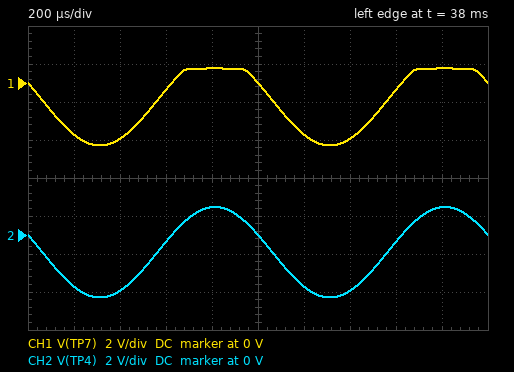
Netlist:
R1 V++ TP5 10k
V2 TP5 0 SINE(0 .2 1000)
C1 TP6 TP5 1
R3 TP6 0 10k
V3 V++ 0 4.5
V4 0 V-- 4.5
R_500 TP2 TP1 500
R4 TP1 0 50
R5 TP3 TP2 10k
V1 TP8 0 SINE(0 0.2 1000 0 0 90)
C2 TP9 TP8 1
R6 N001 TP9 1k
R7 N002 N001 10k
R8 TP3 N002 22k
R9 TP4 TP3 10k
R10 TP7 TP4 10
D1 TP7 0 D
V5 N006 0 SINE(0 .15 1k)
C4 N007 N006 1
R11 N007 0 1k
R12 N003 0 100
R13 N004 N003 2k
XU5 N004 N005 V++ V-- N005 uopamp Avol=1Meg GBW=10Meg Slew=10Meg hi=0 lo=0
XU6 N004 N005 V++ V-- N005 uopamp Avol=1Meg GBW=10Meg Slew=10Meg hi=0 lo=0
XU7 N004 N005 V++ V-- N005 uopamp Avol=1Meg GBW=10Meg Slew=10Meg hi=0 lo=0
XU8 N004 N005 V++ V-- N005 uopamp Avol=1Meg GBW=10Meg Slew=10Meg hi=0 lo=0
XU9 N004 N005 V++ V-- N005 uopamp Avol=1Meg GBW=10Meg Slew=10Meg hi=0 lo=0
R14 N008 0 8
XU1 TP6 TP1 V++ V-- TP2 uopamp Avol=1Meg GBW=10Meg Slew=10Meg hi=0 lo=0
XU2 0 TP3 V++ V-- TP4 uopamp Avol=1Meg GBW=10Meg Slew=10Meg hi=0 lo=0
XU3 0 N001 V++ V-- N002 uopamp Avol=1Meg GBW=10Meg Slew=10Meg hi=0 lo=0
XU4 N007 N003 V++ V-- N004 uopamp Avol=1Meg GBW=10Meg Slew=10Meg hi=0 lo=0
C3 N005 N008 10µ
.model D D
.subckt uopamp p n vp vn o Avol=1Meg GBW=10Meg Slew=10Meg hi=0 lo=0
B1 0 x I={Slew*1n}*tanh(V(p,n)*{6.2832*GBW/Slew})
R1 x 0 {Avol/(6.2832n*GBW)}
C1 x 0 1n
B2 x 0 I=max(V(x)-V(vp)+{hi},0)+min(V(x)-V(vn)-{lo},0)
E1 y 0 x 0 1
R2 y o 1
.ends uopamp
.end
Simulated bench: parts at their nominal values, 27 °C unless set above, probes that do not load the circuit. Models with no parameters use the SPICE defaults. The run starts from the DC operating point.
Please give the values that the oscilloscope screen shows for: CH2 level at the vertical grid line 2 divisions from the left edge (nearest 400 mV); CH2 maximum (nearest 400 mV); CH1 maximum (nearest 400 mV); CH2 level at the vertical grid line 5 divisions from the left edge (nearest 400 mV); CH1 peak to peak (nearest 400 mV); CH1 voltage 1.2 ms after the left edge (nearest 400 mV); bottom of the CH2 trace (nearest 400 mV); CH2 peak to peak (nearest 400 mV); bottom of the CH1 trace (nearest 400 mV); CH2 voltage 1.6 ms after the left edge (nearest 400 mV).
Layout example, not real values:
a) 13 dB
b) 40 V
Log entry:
a) -2.8 V
b) 1.6 V
c) 800 mV
d) 0 V
e) 4.0 V
f) -2.8 V
g) -3.2 V
h) 4.8 V
i) -3.2 V
j) -400 mV
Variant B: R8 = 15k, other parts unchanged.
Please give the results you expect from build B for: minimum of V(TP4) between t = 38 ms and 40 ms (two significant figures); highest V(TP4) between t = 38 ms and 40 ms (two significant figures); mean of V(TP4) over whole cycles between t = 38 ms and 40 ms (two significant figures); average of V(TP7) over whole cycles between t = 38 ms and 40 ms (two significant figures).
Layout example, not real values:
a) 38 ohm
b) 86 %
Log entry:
a) -3.9 V
b) 1.2 V
c) -1.3 V
d) -1.4 V
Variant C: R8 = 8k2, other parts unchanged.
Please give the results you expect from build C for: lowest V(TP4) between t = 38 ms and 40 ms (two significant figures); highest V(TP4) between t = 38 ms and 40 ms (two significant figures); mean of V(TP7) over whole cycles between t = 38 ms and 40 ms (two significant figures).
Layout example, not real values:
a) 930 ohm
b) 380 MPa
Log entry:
a) -4.5 V
b) 850 mV
c) -2.2 V
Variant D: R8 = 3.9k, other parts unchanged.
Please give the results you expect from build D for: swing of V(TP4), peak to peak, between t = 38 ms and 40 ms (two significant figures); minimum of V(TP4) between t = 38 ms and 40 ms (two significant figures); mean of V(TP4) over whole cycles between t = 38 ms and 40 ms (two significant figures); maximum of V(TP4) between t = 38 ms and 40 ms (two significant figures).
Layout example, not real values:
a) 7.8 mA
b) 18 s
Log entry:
a) 5.0 V
b) -4.5 V
c) -3.0 V
d) 450 mV
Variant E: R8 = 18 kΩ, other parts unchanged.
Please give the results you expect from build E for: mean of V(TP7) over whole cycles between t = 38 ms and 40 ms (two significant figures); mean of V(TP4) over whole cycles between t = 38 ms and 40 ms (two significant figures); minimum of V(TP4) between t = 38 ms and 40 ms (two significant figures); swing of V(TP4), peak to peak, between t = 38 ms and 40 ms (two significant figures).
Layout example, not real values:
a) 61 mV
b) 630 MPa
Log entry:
a) -1.2 V
b) -1.1 V
c) -3.6 V
d) 4.9 V
